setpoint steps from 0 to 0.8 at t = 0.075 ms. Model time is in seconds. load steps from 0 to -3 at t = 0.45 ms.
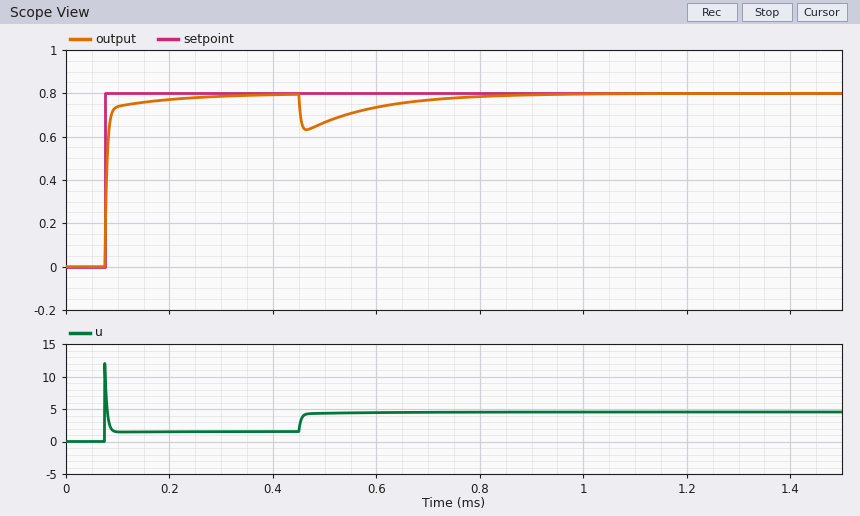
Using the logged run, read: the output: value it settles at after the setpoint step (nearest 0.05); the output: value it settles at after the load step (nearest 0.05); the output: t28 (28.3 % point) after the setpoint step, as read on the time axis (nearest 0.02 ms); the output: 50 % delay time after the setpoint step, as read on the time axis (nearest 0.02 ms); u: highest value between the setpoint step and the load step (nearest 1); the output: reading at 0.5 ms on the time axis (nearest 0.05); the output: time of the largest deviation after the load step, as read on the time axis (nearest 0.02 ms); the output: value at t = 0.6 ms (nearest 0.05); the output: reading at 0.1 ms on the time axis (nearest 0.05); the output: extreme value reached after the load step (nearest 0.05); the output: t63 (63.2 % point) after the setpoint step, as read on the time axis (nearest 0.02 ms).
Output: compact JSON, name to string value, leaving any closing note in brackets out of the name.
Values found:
{"the output: value it settles at after the setpoint step": "0.80", "the output: value it settles at after the load step": "0.80", "the output: t28 (28.3 % point) after the setpoint step, as read on the time axis": "0.08 ms", "the output: 50 % delay time after the setpoint step, as read on the time axis": "0.08 ms", "u: highest value between the setpoint step and the load step": "12", "the output: reading at 0.5 ms on the time axis": "0.65", "the output: time of the largest deviation after the load step, as read on the time axis": "0.46 ms", "the output: value at t = 0.6 ms": "0.75", "the output: reading at 0.1 ms on the time axis": "0.75", "the output: extreme value reached after the load step": "0.65", "the output: t63 (63.2 % point) after the setpoint step, as read on the time axis": "0.08 ms"}
